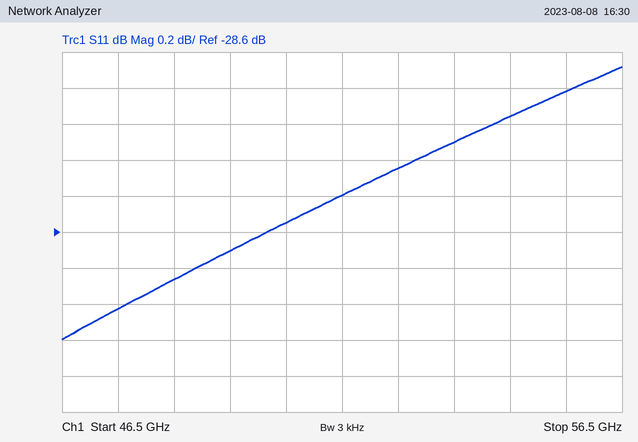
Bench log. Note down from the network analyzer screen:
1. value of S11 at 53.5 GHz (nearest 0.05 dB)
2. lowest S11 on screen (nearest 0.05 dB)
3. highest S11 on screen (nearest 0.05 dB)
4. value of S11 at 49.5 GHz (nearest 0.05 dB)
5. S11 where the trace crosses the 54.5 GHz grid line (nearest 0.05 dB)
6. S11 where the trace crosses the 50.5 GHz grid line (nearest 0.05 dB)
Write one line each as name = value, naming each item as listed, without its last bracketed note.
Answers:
value of S11 at 53.5 GHz = -28.10 dB
lowest S11 on screen = -29.20 dB
highest S11 on screen = -27.70 dB
value of S11 at 49.5 GHz = -28.70 dB
S11 where the trace crosses the 54.5 GHz grid line = -27.95 dB
S11 where the trace crosses the 50.5 GHz grid line = -28.55 dB
